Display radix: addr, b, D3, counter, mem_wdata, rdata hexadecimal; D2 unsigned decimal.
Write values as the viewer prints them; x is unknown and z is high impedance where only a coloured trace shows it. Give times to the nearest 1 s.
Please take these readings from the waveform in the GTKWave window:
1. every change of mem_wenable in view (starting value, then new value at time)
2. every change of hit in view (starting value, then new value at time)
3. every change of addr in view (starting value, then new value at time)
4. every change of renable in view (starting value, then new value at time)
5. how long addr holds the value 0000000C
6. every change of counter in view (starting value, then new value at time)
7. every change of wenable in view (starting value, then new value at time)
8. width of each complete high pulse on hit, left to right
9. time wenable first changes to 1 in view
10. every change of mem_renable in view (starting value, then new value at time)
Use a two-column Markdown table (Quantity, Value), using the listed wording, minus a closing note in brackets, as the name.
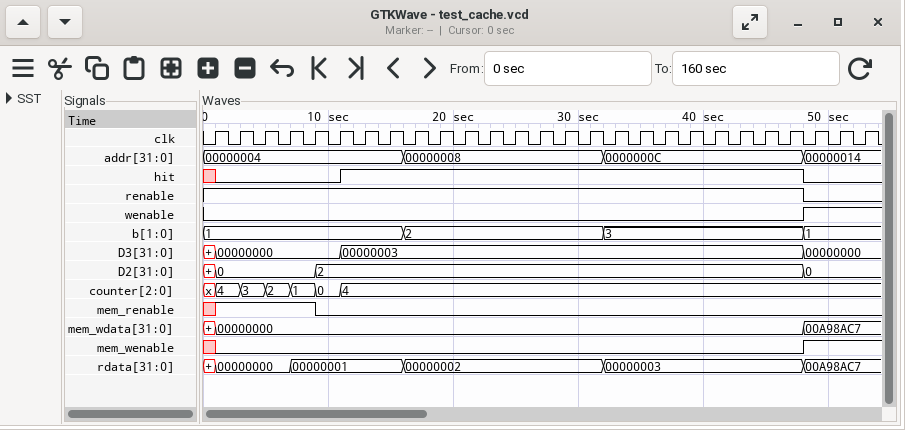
| Quantity | Value |
|---|---|
| every change of mem_wenable in view | x, 0 at 1 s, 1 at 48 s |
| every change of hit in view | x, 0 at 1 s, 1 at 11 s, 0 at 48 s |
| every change of addr in view | 00000004, 00000008 at 16 s, 0000000C at 32 s, 00000014 at 48 s |
| every change of renable in view | 1, 0 at 48 s |
| how long addr holds the value 0000000C | 16 s |
| every change of counter in view | x, 4 at 1 s, 3 at 3 s, 2 at 5 s, 1 at 7 s, 0 at 9 s, 4 at 11 s |
| every change of wenable in view | 0, 1 at 48 s |
| width of each complete high pulse on hit, left to right | 37 s |
| time wenable first changes to 1 in view | 48 s |
| every change of mem_renable in view | x, 1 at 1 s, 0 at 9 s |
